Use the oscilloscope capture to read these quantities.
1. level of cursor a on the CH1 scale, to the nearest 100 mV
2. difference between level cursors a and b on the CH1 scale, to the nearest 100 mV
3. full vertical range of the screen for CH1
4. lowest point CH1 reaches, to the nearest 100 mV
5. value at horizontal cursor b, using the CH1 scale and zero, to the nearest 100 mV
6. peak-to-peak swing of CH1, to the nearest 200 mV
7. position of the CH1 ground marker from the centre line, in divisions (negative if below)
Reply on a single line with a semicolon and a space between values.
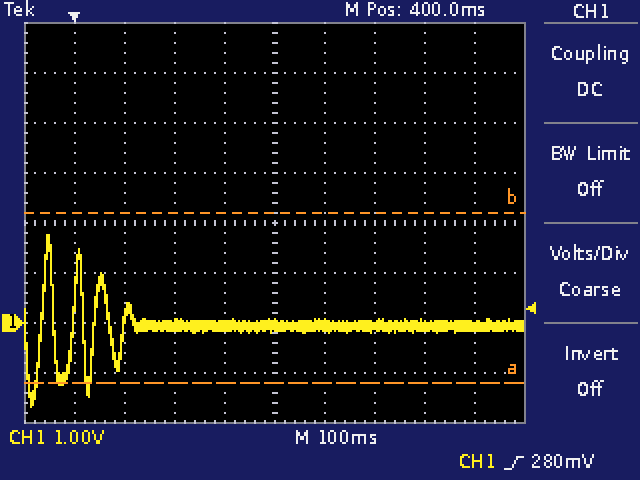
-1.2 V; 3.4 V; 8 V; -1.7 V; 2.2 V; 3.4 V; -2.0 div
